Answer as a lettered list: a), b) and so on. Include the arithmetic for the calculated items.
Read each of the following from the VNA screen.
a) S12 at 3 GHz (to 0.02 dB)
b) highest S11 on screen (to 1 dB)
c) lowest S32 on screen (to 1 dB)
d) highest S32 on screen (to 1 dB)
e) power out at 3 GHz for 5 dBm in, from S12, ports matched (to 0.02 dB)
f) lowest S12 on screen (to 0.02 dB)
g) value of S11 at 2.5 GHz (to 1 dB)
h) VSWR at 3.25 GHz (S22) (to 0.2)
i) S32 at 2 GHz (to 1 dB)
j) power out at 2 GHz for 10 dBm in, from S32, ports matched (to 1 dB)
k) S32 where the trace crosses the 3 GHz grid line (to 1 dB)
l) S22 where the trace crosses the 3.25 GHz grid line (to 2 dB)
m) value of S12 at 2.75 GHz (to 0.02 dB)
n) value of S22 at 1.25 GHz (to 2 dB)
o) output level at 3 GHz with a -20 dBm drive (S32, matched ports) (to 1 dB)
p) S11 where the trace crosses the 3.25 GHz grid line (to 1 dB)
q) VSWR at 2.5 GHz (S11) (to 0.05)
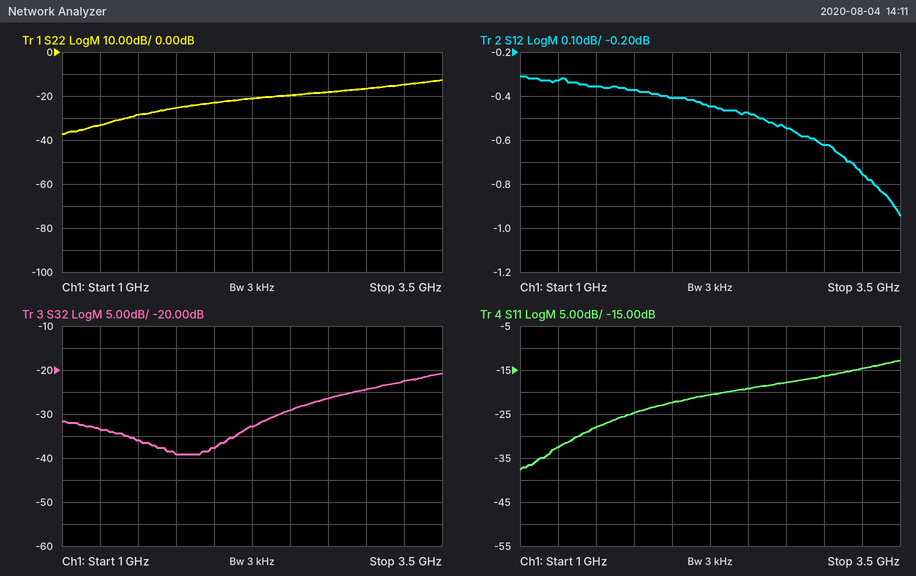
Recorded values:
a) -0.62 dB
b) -13 dB
c) -39 dB
d) -21 dB
e) 5 dBm + (-0.62 dB) = 4.38 dBm
f) -0.94 dB
g) -19 dB
h) |Γ| = 10^(-14/20) = 0.1995; VSWR = (1 + 0.1995)/(1 − 0.1995) ≈ 1.50, so 1.4 to the nearest 0.2
i) -38 dB
j) 10 dBm + (-38 dB) = -28 dBm
k) -24 dB
l) -14 dB
m) -0.54 dB
n) -34 dB
o) -20 dBm + (-24 dB) = -44 dBm
p) -15 dB
q) |Γ| = 10^(-19/20) = 0.1122; VSWR = (1 + 0.1122)/(1 − 0.1122) ≈ 1.25
